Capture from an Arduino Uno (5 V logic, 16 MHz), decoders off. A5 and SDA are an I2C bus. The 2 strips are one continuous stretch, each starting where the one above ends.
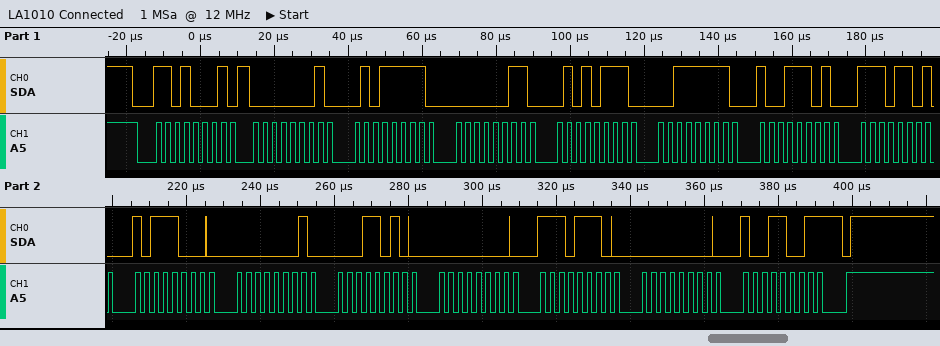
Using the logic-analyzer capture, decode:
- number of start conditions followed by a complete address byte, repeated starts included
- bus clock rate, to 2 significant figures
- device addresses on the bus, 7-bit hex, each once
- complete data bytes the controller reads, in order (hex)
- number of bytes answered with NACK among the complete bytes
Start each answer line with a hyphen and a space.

- 1
- 400 kHz
- 0x68
- 01 5F 03 57 3F 9D ED B8 01 1A 00 EE 00 99
- 1
